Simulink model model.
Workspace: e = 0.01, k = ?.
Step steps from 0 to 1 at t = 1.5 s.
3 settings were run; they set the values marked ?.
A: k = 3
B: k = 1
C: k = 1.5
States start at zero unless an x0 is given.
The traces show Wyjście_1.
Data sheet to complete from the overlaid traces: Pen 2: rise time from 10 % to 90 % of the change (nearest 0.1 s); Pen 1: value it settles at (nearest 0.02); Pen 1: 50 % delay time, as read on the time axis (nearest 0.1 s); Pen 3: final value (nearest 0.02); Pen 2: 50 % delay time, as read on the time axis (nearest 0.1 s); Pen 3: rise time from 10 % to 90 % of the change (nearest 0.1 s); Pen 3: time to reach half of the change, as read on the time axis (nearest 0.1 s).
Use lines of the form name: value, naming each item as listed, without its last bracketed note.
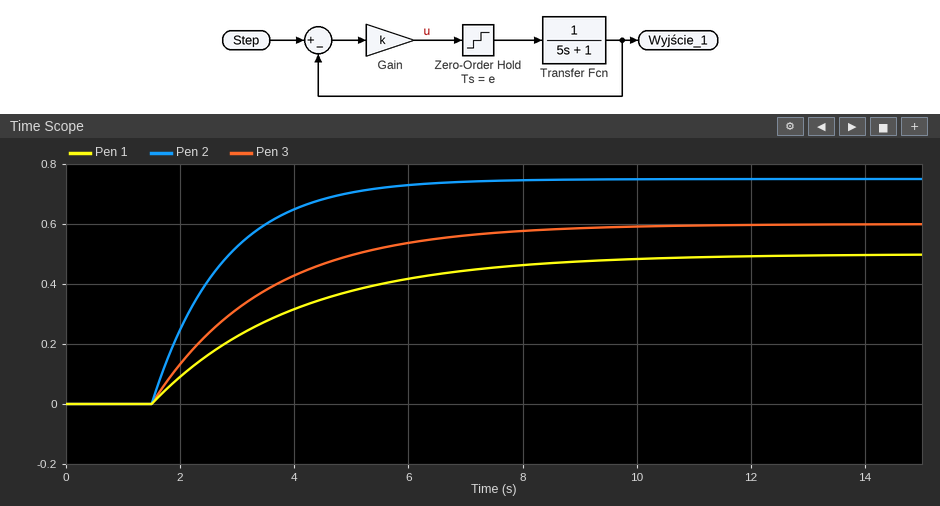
Pen 2: rise time from 10 % to 90 % of the change: 2.7 s
Pen 1: value it settles at: 0.50
Pen 1: 50 % delay time, as read on the time axis: 3.2 s
Pen 3: final value: 0.60
Pen 2: 50 % delay time, as read on the time axis: 2.4 s
Pen 3: rise time from 10 % to 90 % of the change: 4.4 s
Pen 3: time to reach half of the change, as read on the time axis: 2.9 s
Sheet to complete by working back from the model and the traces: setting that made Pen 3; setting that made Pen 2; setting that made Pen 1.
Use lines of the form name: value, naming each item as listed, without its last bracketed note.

setting that made Pen 3: C
setting that made Pen 2: A
setting that made Pen 1: B
